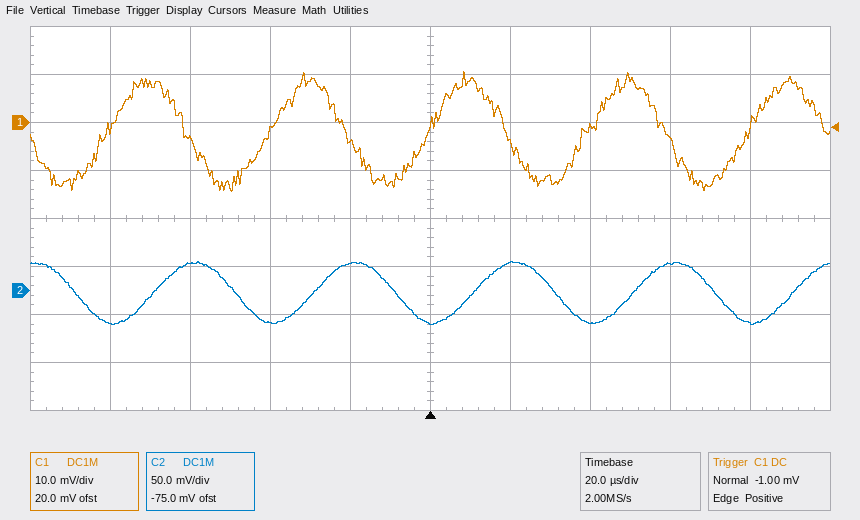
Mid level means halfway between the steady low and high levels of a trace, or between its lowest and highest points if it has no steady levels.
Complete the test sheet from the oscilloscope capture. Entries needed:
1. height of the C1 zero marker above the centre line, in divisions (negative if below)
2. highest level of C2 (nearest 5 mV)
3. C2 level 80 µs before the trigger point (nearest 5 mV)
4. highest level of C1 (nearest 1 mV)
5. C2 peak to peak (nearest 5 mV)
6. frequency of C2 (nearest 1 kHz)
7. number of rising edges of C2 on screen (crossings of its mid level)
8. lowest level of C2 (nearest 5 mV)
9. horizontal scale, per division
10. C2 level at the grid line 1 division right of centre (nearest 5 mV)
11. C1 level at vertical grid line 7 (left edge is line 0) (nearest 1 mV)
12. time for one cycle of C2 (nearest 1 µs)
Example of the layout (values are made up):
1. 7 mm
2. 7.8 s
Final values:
1. +2.0 div
2. 30 mV
3. -35 mV
4. 11 mV
5. 65 mV
6. 25 kHz
7. 5
8. -35 mV
9. 20 µs
10. 30 mV
11. -1 mV
12. 40 µs
